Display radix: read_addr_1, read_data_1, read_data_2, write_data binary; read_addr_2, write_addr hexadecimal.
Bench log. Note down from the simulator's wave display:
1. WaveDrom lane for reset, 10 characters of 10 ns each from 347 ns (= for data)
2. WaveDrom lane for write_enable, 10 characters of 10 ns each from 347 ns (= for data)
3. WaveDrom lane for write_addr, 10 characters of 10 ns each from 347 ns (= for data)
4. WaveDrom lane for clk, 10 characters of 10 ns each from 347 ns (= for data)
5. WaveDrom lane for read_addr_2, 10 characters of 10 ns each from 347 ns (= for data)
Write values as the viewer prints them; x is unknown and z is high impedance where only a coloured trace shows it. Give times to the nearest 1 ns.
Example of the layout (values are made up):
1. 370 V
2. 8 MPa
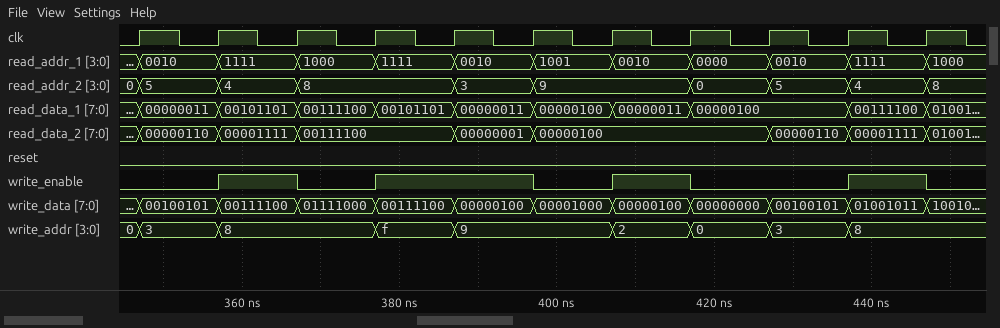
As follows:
1. {name: 'reset', wave: '0.........'}
2. {name: 'write_enable', wave: '0101.010.1'}
3. {name: 'write_addr', wave: '==.==.====', data: '3 8 f 9 2 0 3 8'}
4. {name: 'clk', wave: 'p.........'}
5. {name: 'read_addr_2', wave: '===.==.===', data: '5 4 8 3 9 0 5 4'}
